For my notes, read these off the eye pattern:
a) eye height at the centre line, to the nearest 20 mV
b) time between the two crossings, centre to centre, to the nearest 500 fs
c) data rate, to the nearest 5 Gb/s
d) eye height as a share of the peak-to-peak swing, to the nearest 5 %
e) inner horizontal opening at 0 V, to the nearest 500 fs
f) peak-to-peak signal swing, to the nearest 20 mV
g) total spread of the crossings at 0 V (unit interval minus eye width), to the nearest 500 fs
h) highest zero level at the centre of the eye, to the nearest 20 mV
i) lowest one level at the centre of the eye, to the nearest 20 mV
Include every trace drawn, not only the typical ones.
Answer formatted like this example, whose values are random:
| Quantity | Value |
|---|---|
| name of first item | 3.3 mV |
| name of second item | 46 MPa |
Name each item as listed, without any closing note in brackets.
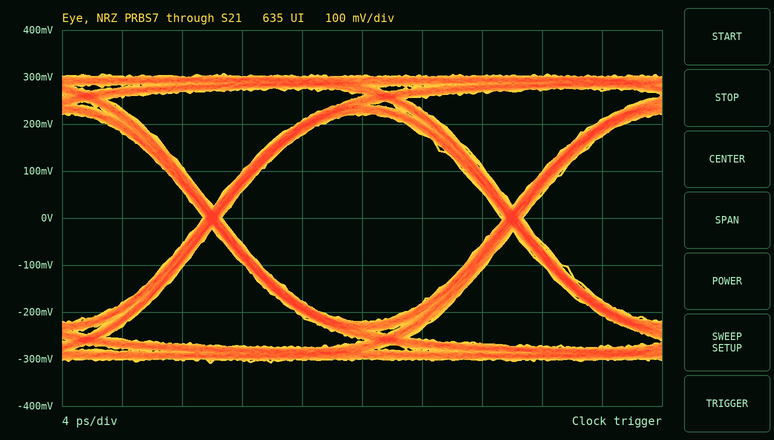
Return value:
| Quantity | Value |
|---|---|
| eye height at the centre line, to the nearest 20 mV | 440 mV |
| time between the two crossings, centre to centre, to the nearest 500 fs | 20.0 ps |
| data rate, to the nearest 5 Gb/s | 50 Gb/s |
| eye height as a share of the peak-to-peak swing, to the nearest 5 % | 70 % |
| inner horizontal opening at 0 V, to the nearest 500 fs | 18.5 ps |
| peak-to-peak signal swing, to the nearest 20 mV | 620 mV |
| total spread of the crossings at 0 V (unit interval minus eye width), to the nearest 500 fs | 1.5 ps |
| highest zero level at the centre of the eye, to the nearest 20 mV | -220 mV |
| lowest one level at the centre of the eye, to the nearest 20 mV | 220 mV |
